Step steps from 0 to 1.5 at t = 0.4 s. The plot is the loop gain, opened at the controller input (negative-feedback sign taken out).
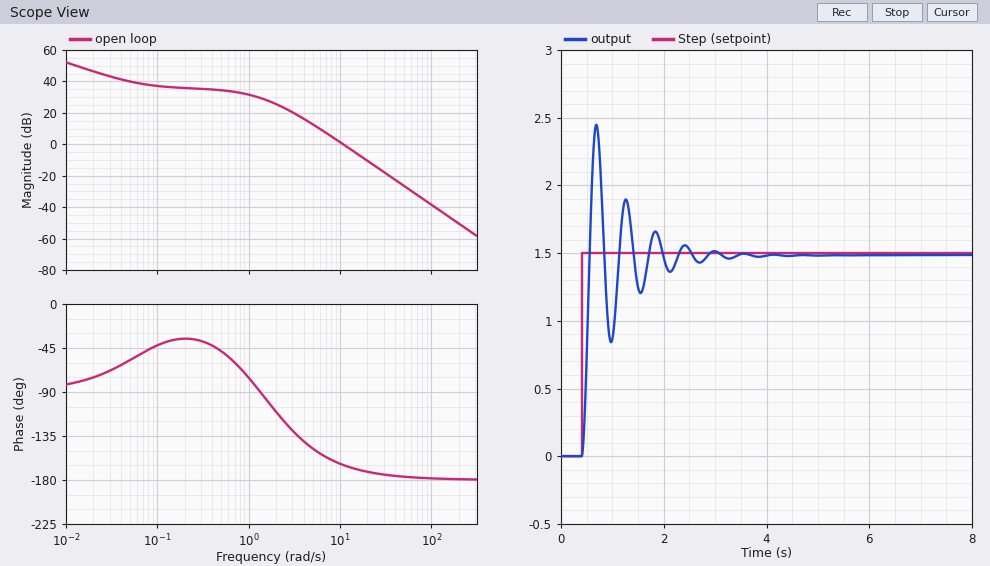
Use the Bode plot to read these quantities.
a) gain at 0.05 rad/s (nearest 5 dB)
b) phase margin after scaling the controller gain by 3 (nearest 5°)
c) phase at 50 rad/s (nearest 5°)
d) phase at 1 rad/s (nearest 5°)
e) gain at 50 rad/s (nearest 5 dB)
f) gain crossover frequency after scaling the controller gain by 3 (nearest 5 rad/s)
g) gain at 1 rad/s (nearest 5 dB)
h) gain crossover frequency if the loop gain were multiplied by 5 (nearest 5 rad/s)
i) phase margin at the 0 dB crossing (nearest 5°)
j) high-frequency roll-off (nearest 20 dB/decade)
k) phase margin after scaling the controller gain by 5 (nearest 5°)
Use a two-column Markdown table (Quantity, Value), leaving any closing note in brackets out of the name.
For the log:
| Quantity | Value |
|---|---|
| gain at 0.05 rad/s | 40 dB |
| phase margin after scaling the controller gain by 3 | 10° |
| phase at 50 rad/s | -175° |
| phase at 1 rad/s | -75° |
| gain at 50 rad/s | -25 dB |
| gain crossover frequency after scaling the controller gain by 3 | 20 rad/s |
| gain at 1 rad/s | 30 dB |
| gain crossover frequency if the loop gain were multiplied by 5 | 25 rad/s |
| phase margin at the 0 dB crossing | 15° |
| high-frequency roll-off | -40 dB/decade |
| phase margin after scaling the controller gain by 5 | 5° |
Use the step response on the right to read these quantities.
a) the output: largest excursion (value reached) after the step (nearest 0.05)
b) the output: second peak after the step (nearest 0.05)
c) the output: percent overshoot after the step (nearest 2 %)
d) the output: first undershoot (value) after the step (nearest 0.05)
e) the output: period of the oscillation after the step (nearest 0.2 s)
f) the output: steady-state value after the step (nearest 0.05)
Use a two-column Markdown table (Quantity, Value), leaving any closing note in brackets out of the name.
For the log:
| Quantity | Value |
|---|---|
| the output: largest excursion (value reached) after the step | 2.45 |
| the output: second peak after the step | 1.90 |
| the output: percent overshoot after the step | 64 % |
| the output: first undershoot (value) after the step | 0.85 |
| the output: period of the oscillation after the step | 0.6 s |
| the output: steady-state value after the step | 1.50 |
